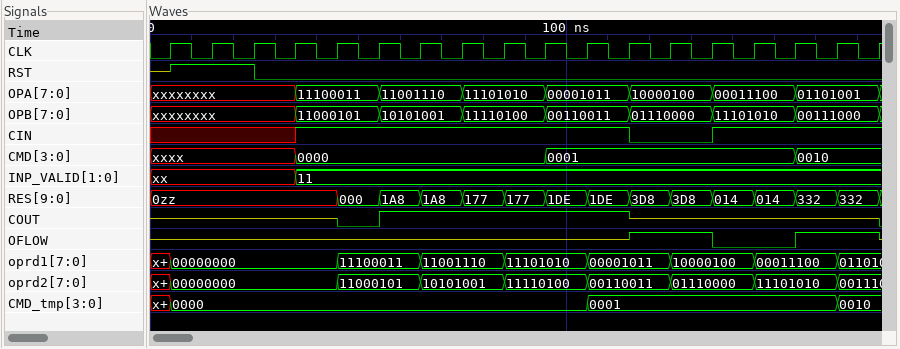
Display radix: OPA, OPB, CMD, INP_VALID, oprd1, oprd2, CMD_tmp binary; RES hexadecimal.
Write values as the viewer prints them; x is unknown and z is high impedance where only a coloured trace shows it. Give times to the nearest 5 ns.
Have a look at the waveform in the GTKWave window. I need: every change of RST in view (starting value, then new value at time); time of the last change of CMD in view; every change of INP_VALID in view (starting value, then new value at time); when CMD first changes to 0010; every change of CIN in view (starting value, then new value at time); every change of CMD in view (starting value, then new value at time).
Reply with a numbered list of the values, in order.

1. z, 1 at 5 ns, 0 at 25 ns
2. 155 ns
3. xx, 11 at 35 ns
4. 155 ns
5. x, 1 at 35 ns, 0 at 115 ns, 1 at 135 ns
6. xxxx, 0000 at 35 ns, 0001 at 95 ns, 0010 at 155 ns
